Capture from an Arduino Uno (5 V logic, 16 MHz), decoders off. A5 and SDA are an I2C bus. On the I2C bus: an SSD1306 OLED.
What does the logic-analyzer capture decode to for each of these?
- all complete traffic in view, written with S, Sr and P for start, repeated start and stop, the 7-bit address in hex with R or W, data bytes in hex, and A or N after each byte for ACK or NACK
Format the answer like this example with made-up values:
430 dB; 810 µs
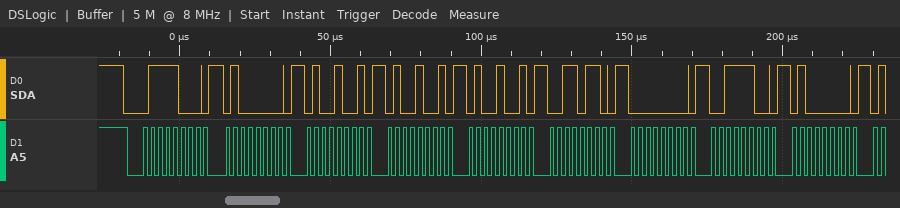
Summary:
S 3CW A 40 A 49 A 49 A 49 A 36 A 00 A 3C A 40 A
